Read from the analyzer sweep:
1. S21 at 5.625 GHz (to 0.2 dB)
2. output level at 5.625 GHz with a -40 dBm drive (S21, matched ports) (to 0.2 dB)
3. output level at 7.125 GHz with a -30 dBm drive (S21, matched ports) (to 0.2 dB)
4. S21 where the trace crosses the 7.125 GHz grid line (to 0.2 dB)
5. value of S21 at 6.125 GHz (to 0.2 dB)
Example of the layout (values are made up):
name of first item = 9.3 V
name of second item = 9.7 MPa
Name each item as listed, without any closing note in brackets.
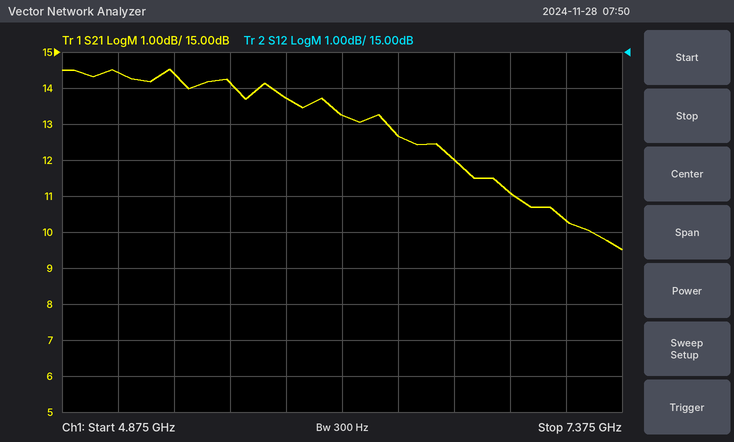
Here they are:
S21 at 5.625 GHz = 14.2 dB
output level at 5.625 GHz with a -40 dBm drive (S21, matched ports) = -25.8 dBm
output level at 7.125 GHz with a -30 dBm drive (S21, matched ports) = -19.6 dBm
S21 where the trace crosses the 7.125 GHz grid line = 10.4 dB
value of S21 at 6.125 GHz = 13.2 dB
